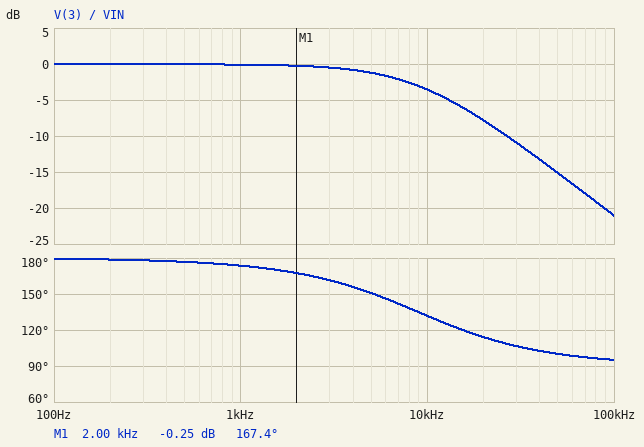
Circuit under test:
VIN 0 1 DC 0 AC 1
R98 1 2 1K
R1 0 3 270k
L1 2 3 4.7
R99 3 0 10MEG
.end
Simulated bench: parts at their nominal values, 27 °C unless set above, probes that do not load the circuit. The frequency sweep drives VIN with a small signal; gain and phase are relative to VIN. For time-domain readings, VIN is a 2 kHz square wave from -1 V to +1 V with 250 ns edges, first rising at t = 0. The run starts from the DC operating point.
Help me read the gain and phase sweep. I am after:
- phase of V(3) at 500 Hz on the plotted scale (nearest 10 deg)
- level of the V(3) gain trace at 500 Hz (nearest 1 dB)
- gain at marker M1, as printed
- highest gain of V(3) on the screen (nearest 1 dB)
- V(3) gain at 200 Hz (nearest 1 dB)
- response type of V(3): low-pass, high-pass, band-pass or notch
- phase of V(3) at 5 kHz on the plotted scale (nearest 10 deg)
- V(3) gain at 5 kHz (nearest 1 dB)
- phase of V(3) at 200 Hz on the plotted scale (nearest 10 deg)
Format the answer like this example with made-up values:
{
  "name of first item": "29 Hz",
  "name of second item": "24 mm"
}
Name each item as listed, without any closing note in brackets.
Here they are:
{
  "phase of V(3) at 500 Hz on the plotted scale": "180 deg",
  "level of the V(3) gain trace at 500 Hz": "0 dB",
  "gain at marker M1, as printed": "-0.25 dB",
  "highest gain of V(3) on the screen": "0 dB",
  "V(3) gain at 200 Hz": "0 dB",
  "response type of V(3): low-pass, high-pass, band-pass or notch": "low-pass",
  "phase of V(3) at 5 kHz on the plotted scale": "150 deg",
  "V(3) gain at 5 kHz": "-1 dB",
  "phase of V(3) at 200 Hz on the plotted scale": "180 deg"
}
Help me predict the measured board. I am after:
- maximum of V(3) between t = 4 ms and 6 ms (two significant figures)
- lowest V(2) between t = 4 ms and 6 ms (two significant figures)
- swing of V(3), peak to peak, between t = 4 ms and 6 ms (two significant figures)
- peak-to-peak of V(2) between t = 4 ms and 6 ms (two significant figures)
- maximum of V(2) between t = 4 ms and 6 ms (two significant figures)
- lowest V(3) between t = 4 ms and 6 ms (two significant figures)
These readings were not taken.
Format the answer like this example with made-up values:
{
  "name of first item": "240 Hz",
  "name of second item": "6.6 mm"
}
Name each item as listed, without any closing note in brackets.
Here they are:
{
  "maximum of V(3) between t = 4 ms and 6 ms": "1.0 V",
  "lowest V(2) between t = 4 ms and 6 ms": "-1.0 V",
  "swing of V(3), peak to peak, between t = 4 ms and 6 ms": "2.0 V",
  "peak-to-peak of V(2) between t = 4 ms and 6 ms": "2.0 V",
  "maximum of V(2) between t = 4 ms and 6 ms": "1.0 V",
  "lowest V(3) between t = 4 ms and 6 ms": "-1.0 V"
}
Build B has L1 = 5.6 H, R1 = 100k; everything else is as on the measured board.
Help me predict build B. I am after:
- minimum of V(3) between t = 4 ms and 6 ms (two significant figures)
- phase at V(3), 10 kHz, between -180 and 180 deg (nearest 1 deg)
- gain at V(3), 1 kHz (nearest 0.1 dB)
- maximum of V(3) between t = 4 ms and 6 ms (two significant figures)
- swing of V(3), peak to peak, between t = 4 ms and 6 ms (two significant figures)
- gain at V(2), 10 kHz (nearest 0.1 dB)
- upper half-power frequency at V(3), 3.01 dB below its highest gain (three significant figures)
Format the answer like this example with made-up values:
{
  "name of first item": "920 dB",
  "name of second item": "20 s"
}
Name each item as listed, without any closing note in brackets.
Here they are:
{
  "minimum of V(3) between t = 4 ms and 6 ms": "-970 mV",
  "phase at V(3), 10 kHz, between -180 and 180 deg": "106 deg",
  "gain at V(3), 1 kHz": "-0.6 dB",
  "maximum of V(3) between t = 4 ms and 6 ms": "970 mV",
  "swing of V(3), peak to peak, between t = 4 ms and 6 ms": "1.9 V",
  "gain at V(2), 10 kHz": "0 dB",
  "upper half-power frequency at V(3), 3.01 dB below its highest gain": "2.84 kHz"
}
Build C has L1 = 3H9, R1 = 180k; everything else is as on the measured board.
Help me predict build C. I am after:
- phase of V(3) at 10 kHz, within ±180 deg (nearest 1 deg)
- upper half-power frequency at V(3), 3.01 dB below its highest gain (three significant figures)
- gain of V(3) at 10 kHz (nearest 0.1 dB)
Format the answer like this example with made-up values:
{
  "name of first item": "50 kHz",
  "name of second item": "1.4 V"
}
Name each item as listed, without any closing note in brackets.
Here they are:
{
  "phase of V(3) at 10 kHz, within ±180 deg": "126 deg",
  "upper half-power frequency at V(3), 3.01 dB below its highest gain": "7.26 kHz",
  "gain of V(3) at 10 kHz": "-4.7 dB"
}
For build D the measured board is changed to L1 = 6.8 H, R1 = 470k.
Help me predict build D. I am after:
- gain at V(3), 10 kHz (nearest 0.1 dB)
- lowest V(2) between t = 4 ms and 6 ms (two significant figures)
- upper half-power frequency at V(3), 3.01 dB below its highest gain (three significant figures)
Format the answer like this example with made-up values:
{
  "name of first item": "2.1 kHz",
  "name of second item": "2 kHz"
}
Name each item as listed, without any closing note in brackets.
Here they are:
{
  "gain at V(3), 10 kHz": "-2.8 dB",
  "lowest V(2) between t = 4 ms and 6 ms": "-1.0 V",
  "upper half-power frequency at V(3), 3.01 dB below its highest gain": "10.5 kHz"
}
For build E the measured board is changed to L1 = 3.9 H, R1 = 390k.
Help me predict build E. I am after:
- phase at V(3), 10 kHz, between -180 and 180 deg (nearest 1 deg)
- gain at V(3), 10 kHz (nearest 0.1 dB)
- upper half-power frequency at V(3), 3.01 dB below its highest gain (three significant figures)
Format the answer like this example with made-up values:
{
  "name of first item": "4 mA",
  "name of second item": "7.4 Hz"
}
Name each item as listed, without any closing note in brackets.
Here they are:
{
  "phase at V(3), 10 kHz, between -180 and 180 deg": "147 deg",
  "gain at V(3), 10 kHz": "-1.6 dB",
  "upper half-power frequency at V(3), 3.01 dB below its highest gain": "15.4 kHz"
}
